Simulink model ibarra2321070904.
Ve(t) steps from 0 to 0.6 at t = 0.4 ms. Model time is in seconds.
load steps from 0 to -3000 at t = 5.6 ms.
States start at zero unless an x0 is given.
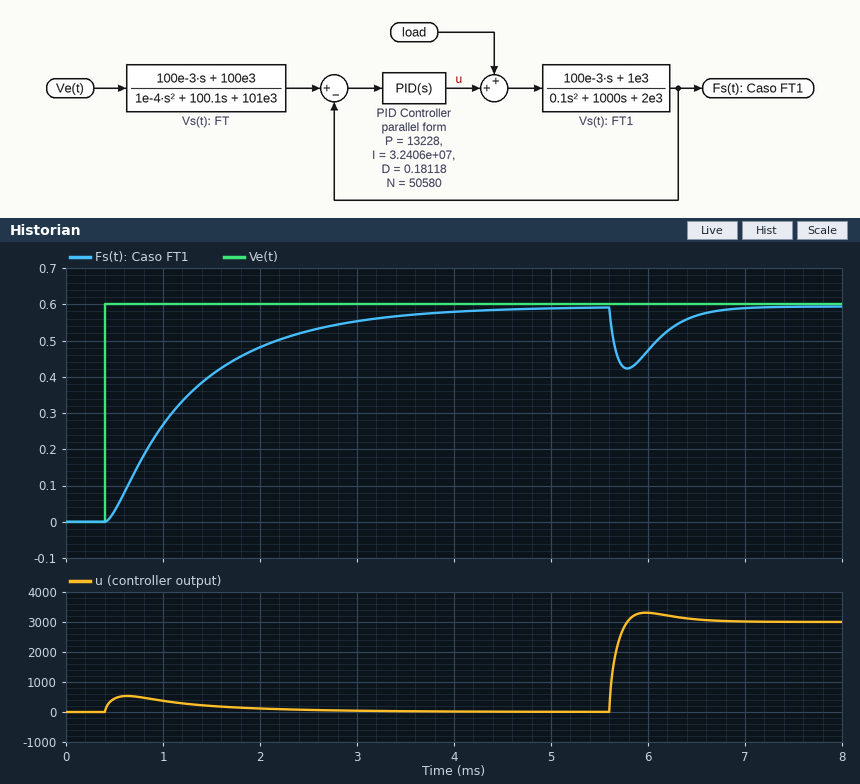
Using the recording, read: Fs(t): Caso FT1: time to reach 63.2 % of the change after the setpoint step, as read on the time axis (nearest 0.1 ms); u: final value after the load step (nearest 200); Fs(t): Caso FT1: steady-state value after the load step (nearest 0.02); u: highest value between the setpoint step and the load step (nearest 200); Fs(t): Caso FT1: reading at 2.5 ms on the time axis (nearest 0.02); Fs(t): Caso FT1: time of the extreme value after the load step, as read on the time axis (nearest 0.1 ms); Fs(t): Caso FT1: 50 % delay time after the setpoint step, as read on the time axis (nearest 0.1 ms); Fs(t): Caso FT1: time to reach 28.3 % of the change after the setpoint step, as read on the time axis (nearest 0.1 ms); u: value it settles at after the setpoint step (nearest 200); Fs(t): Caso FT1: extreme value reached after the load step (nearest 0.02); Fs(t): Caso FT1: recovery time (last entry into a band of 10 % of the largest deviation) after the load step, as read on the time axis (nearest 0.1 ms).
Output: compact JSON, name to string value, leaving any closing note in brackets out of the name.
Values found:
{"Fs(t): Caso FT1: time to reach 63.2 % of the change after the setpoint step, as read on the time axis": "1.4 ms", "u: final value after the load step": "3000", "Fs(t): Caso FT1: steady-state value after the load step": "0.60", "u: highest value between the setpoint step and the load step": "600", "Fs(t): Caso FT1: reading at 2.5 ms on the time axis": "0.52", "Fs(t): Caso FT1: time of the extreme value after the load step, as read on the time axis": "5.8 ms", "Fs(t): Caso FT1: 50 % delay time after the setpoint step, as read on the time axis": "1.1 ms", "Fs(t): Caso FT1: time to reach 28.3 % of the change after the setpoint step, as read on the time axis": "0.8 ms", "u: value it settles at after the setpoint step": "0", "Fs(t): Caso FT1: extreme value reached after the load step": "0.42", "Fs(t): Caso FT1: recovery time (last entry into a band of 10 % of the largest deviation) after the load step, as read on the time axis": "6.6 ms"}
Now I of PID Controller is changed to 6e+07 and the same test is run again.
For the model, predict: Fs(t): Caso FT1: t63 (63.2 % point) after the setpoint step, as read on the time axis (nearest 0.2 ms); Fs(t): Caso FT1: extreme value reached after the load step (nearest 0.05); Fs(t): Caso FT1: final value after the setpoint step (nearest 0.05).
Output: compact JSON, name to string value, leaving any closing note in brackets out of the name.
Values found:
{"Fs(t): Caso FT1: t63 (63.2 % point) after the setpoint step, as read on the time axis": "1.4 ms", "Fs(t): Caso FT1: extreme value reached after the load step": "0.45", "Fs(t): Caso FT1: final value after the setpoint step": "0.60"}
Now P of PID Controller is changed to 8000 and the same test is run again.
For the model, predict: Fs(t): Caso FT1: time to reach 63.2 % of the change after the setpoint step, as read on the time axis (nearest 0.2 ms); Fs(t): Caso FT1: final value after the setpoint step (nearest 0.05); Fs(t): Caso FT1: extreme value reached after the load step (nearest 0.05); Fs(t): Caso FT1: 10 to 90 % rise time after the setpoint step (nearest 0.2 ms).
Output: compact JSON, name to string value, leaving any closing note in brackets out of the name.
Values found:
{"Fs(t): Caso FT1: time to reach 63.2 % of the change after the setpoint step, as read on the time axis": "1.4 ms", "Fs(t): Caso FT1: final value after the setpoint step": "0.60", "Fs(t): Caso FT1: extreme value reached after the load step": "0.35", "Fs(t): Caso FT1: 10 to 90 % rise time after the setpoint step": "2.0 ms"}
